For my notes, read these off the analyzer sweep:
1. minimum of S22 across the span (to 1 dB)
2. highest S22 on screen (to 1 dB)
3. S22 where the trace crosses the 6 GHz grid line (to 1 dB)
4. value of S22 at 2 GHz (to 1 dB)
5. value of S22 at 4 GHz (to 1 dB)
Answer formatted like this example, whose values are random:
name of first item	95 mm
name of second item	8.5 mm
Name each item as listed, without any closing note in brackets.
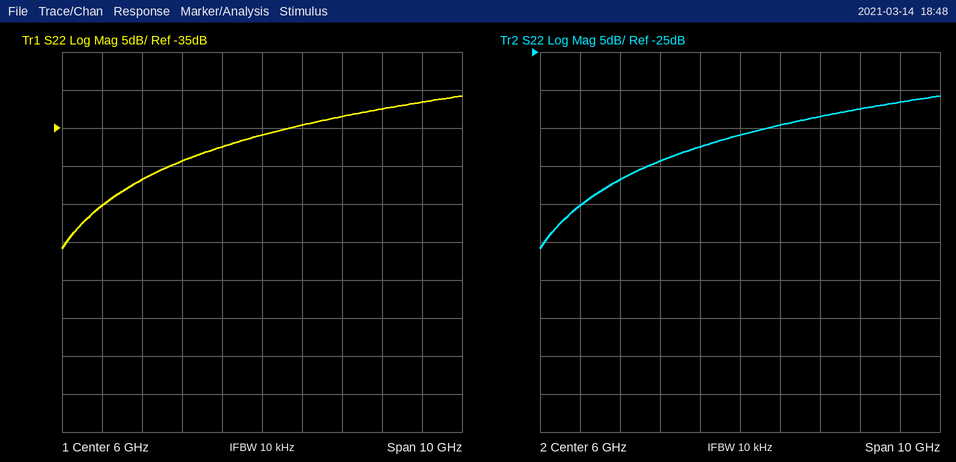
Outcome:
minimum of S22 across the span	-51 dB
highest S22 on screen	-31 dB
S22 where the trace crosses the 6 GHz grid line	-36 dB
value of S22 at 2 GHz	-45 dB
value of S22 at 4 GHz	-39 dB
